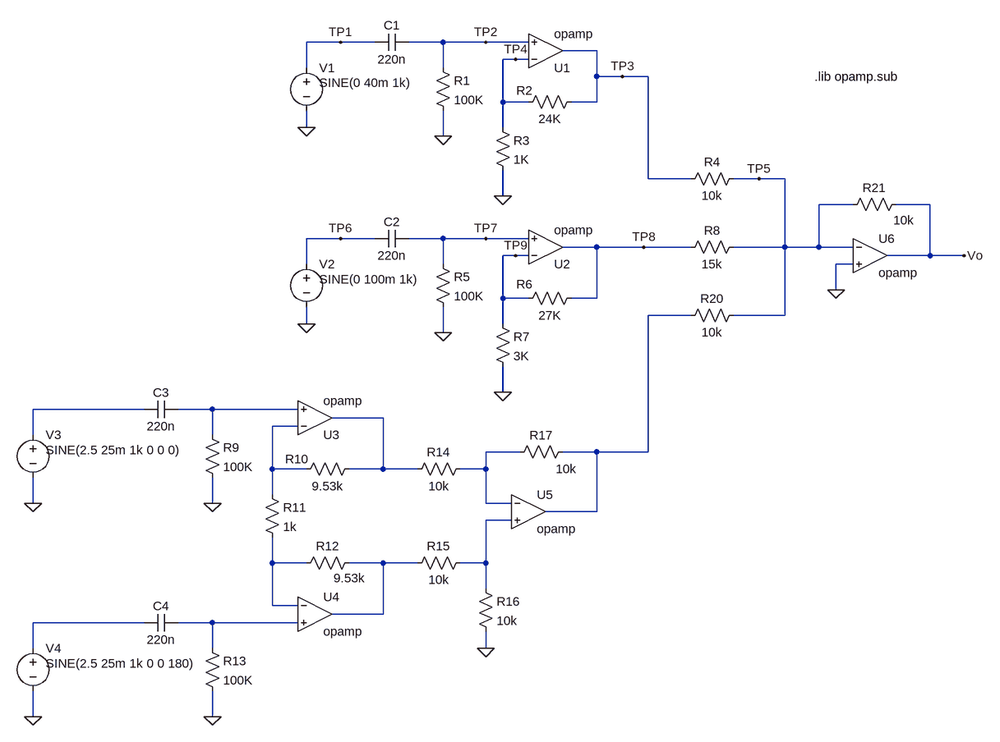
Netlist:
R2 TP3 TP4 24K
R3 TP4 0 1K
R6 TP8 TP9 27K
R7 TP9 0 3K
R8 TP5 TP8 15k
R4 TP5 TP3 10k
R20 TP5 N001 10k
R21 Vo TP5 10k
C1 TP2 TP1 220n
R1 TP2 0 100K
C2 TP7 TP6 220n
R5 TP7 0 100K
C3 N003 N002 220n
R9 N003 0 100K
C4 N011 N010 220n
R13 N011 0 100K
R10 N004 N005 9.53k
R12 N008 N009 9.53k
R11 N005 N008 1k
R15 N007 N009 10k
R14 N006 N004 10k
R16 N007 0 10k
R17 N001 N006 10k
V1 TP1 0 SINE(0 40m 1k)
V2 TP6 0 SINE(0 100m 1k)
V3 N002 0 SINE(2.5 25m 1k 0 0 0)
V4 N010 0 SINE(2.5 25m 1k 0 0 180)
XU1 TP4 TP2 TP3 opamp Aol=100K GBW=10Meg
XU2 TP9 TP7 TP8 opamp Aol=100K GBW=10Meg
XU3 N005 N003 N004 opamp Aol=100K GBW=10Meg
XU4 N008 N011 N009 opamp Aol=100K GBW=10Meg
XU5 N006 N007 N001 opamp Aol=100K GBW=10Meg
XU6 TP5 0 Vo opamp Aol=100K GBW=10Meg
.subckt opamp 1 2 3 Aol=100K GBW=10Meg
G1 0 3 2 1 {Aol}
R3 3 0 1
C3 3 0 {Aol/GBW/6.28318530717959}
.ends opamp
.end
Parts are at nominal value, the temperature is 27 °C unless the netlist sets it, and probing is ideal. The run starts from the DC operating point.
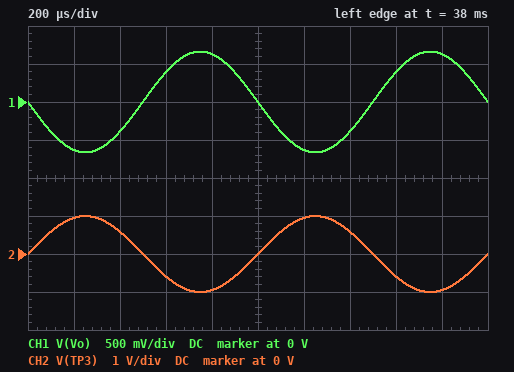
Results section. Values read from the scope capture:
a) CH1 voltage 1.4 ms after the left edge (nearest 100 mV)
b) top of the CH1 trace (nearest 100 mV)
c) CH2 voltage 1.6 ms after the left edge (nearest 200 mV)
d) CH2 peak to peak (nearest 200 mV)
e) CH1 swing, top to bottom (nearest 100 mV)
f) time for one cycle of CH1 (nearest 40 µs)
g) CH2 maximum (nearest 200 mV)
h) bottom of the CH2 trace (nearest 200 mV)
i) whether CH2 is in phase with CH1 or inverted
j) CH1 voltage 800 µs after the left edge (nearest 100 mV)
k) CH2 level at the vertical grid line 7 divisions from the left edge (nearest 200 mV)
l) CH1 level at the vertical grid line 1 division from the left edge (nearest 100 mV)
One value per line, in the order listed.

-400 mV
700 mV
-600 mV
2.0 V
1.3 V
1.00 ms
1.0 V
-1.0 V
inverted
600 mV
600 mV
-600 mV
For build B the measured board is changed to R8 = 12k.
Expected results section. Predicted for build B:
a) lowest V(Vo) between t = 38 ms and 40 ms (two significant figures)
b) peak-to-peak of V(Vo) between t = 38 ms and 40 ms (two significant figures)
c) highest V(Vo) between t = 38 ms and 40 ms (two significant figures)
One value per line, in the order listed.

-830 mV
1.7 V
830 mV
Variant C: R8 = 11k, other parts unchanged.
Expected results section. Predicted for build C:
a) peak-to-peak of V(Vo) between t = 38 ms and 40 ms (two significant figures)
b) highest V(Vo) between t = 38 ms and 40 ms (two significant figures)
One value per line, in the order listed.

1.8 V
910 mV
